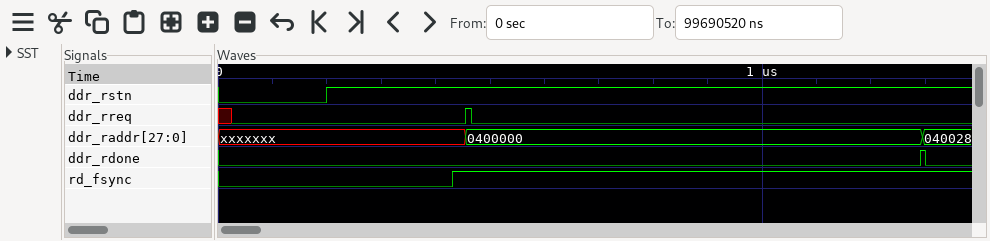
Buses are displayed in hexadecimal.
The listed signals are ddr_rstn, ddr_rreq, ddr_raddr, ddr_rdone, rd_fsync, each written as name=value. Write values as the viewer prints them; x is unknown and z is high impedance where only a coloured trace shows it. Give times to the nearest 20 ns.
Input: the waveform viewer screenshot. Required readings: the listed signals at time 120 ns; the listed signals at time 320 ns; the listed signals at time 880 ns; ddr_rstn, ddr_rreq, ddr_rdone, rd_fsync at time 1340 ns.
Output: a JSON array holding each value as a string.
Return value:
["ddr_rstn=0, ddr_rreq=0, ddr_raddr=xxxxxxx, ddr_rdone=0, rd_fsync=0", "ddr_rstn=1, ddr_rreq=0, ddr_raddr=xxxxxxx, ddr_rdone=0, rd_fsync=0", "ddr_rstn=1, ddr_rreq=0, ddr_raddr=0400000, ddr_rdone=0, rd_fsync=1", "ddr_rstn=1, ddr_rreq=0, ddr_rdone=0, rd_fsync=1"]
